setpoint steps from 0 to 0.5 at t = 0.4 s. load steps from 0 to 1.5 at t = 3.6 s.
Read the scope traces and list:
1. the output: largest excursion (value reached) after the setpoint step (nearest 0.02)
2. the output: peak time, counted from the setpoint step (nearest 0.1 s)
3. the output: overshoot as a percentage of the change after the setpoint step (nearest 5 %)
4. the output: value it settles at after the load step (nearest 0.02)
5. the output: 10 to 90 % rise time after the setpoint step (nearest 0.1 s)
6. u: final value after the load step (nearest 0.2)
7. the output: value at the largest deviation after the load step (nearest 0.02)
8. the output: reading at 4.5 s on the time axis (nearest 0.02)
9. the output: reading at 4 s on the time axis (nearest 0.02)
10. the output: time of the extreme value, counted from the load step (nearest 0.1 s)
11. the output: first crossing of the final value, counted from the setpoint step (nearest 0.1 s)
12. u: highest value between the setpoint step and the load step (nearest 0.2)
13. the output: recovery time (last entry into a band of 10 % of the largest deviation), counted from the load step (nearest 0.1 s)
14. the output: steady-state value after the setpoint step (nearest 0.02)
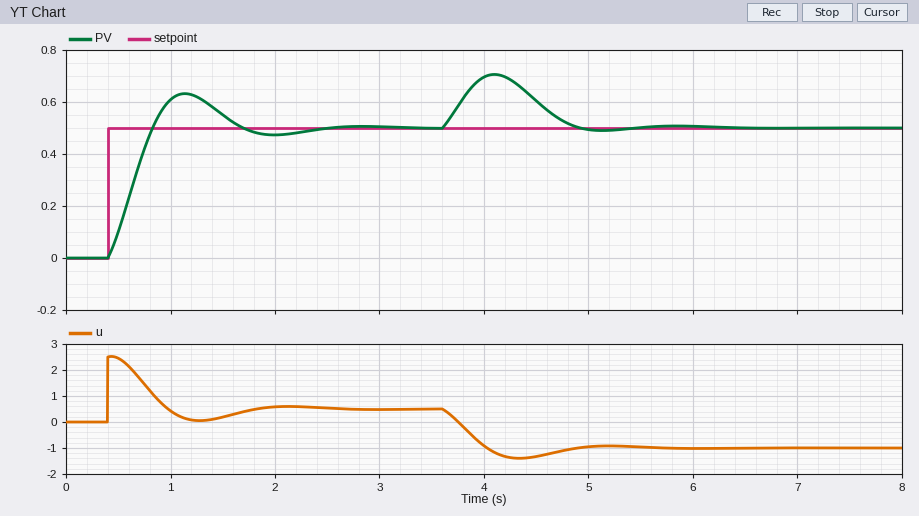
0.64
0.7 s
25 %
0.50
0.3 s
-1.0
0.70
0.60
0.70
0.5 s
0.4 s
2.6
1.2 s
0.50
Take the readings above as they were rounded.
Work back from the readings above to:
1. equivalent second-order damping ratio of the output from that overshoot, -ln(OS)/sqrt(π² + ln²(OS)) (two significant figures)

0.40
